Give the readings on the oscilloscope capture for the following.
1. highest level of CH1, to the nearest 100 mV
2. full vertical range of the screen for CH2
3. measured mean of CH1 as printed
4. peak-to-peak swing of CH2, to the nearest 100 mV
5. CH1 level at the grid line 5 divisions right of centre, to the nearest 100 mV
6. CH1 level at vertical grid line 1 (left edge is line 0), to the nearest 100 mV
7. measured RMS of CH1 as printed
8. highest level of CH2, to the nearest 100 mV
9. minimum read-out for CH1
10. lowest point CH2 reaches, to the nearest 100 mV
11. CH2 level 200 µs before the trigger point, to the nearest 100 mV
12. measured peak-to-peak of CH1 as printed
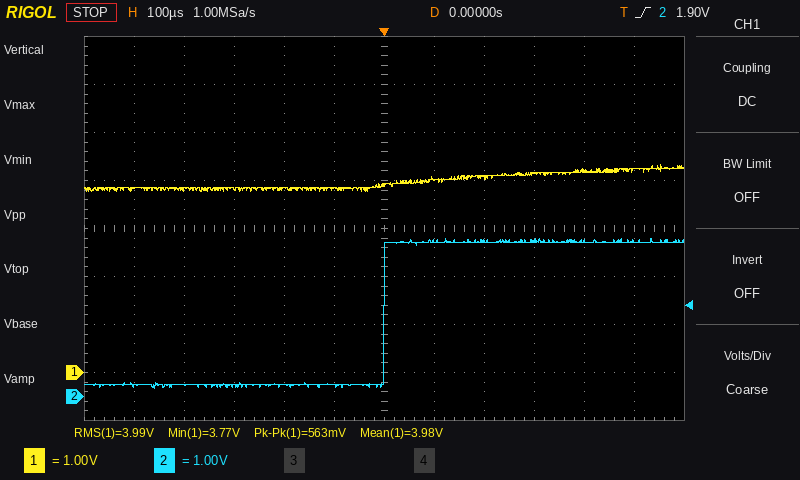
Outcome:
4.3 V
8 V
3.98 V
3.1 V
4.2 V
3.8 V
3.99 V
3.3 V
3.77 V
200 mV
200 mV
563 mV
